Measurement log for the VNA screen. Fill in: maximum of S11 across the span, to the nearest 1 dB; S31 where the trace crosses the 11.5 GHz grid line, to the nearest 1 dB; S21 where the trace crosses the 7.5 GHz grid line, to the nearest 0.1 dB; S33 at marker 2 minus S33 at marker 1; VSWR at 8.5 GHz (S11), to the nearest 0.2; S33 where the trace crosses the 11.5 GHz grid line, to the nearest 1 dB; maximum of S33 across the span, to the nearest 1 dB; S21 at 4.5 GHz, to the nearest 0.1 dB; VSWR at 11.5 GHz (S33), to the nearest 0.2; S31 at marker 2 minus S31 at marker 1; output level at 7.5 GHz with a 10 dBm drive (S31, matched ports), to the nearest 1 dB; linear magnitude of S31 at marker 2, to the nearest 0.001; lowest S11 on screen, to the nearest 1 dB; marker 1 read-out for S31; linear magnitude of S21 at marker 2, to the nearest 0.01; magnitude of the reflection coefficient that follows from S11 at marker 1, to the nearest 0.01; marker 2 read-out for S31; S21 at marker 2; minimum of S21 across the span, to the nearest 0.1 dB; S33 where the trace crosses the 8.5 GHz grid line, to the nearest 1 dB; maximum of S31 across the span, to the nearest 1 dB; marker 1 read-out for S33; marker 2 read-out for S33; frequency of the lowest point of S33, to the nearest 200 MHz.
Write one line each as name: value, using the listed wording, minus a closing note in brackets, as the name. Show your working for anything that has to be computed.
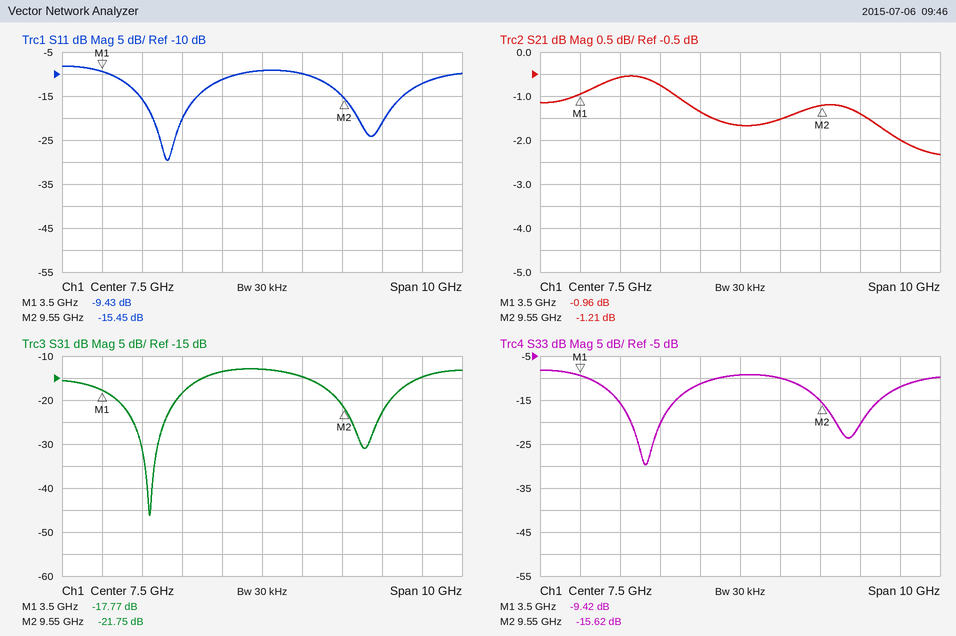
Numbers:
maximum of S11 across the span, to the nearest 1 dB: -8 dB
S31 where the trace crosses the 11.5 GHz grid line, to the nearest 1 dB: -15 dB
S21 where the trace crosses the 7.5 GHz grid line, to the nearest 0.1 dB: -1.7 dB
S33 at marker 2 minus S33 at marker 1: -15.62 − (-9.42) = -6.20 dB
VSWR at 8.5 GHz (S11), to the nearest 0.2: |Γ| = 10^(-10/20) = 0.3162; VSWR = (1 + 0.3162)/(1 − 0.3162) ≈ 1.92, so 2.0 to the nearest 0.2
S33 where the trace crosses the 11.5 GHz grid line, to the nearest 1 dB: -12 dB
maximum of S33 across the span, to the nearest 1 dB: -8 dB
S21 at 4.5 GHz, to the nearest 0.1 dB: -0.6 dB
VSWR at 11.5 GHz (S33), to the nearest 0.2: |Γ| = 10^(-12/20) = 0.2512; VSWR = (1 + 0.2512)/(1 − 0.2512) ≈ 1.67, so 1.6 to the nearest 0.2
S31 at marker 2 minus S31 at marker 1: -21.75 − (-17.77) = -3.98 dB
output level at 7.5 GHz with a 10 dBm drive (S31, matched ports), to the nearest 1 dB: 10 dBm + (-13 dB) = -3 dBm
linear magnitude of S31 at marker 2, to the nearest 0.001: 10^(-21.75/20) ≈ 0.082
lowest S11 on screen, to the nearest 1 dB: -30 dB
marker 1 read-out for S31: -17.77 dB
linear magnitude of S21 at marker 2, to the nearest 0.01: 10^(-1.21/20) ≈ 0.87
magnitude of the reflection coefficient that follows from S11 at marker 1, to the nearest 0.01: 10^(-9.43/20) ≈ 0.34
marker 2 read-out for S31: -21.75 dB
S21 at marker 2: -1.21 dB
minimum of S21 across the span, to the nearest 0.1 dB: -2.3 dB
S33 where the trace crosses the 8.5 GHz grid line, to the nearest 1 dB: -10 dB
maximum of S31 across the span, to the nearest 1 dB: -13 dB
marker 1 read-out for S33: -9.42 dB
marker 2 read-out for S33: -15.62 dB
frequency of the lowest point of S33, to the nearest 200 MHz: 5.2 GHz
